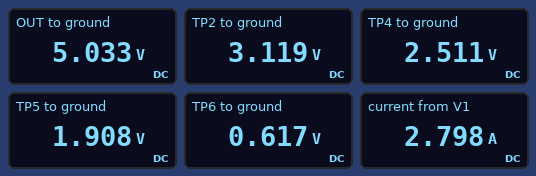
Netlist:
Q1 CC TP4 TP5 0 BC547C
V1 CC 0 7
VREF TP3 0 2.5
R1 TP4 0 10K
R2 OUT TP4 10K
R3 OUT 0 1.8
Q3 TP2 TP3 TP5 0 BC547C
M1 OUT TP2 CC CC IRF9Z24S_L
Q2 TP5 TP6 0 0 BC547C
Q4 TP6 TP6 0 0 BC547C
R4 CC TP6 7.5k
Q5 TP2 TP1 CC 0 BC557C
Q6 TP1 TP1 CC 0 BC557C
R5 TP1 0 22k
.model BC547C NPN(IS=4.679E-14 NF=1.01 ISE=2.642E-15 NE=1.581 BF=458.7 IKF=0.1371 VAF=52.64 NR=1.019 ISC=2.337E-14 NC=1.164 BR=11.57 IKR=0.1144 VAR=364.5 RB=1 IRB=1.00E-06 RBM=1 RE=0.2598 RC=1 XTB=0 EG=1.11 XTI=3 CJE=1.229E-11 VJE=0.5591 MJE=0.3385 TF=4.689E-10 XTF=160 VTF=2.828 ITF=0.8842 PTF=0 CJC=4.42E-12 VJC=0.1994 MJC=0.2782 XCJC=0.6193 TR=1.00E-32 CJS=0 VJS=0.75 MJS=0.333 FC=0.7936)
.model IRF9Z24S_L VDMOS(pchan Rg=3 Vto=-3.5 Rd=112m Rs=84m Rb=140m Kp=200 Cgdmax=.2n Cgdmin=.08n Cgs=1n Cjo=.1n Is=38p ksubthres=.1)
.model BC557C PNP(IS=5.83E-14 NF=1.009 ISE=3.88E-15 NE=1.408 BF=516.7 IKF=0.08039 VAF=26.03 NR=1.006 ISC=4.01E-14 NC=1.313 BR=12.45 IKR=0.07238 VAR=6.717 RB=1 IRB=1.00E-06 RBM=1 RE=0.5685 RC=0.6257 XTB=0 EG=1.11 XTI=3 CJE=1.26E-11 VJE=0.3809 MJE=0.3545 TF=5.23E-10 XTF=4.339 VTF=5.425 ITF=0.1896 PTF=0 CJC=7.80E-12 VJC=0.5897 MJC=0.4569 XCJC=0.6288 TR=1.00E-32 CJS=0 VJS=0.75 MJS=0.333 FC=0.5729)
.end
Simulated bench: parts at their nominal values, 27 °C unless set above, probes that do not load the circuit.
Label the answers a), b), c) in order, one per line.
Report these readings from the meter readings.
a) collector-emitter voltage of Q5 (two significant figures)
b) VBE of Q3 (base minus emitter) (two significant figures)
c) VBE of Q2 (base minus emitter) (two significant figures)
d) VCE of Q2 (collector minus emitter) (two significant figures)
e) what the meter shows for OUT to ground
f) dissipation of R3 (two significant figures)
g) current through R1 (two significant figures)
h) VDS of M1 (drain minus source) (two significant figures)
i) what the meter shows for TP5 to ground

a) -3.9 V
b) 590 mV
c) 620 mV
d) 1.9 V
e) 5.033 V
f) 14 W
g) 250 µA
h) -2.0 V
i) 1.908 V
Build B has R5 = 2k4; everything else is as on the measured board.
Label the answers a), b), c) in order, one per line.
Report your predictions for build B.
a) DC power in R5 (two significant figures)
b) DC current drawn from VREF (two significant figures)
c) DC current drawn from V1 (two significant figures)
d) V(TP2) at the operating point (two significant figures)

a) 17 mW
b) 1.8 µA
c) 4.4 mA
d) 7.0 V
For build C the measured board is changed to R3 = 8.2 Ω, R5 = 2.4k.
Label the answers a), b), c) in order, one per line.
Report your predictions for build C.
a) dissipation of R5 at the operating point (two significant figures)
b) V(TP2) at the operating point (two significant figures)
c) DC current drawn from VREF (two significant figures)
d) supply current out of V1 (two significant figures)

a) 17 mW
b) 7.0 V
c) 1.8 µA
d) 4.4 mA
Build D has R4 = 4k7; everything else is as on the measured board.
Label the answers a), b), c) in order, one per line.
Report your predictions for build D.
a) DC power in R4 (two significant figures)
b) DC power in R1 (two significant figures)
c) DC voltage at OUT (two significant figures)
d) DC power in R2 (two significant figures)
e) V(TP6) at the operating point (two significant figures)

a) 8.6 mW
b) 640 µW
c) 5.1 V
d) 650 µW
e) 630 mV
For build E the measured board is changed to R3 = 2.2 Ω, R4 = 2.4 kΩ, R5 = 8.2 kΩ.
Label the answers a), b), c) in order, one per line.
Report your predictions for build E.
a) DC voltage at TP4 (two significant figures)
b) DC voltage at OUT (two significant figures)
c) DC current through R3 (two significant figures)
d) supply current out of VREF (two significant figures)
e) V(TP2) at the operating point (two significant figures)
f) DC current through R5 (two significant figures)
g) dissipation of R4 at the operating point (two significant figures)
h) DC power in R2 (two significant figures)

a) 2.5 V
b) 5.1 V
c) 2.3 A
d) 1.9 µA
e) 3.2 V
f) 780 µA
g) 17 mW
h) 650 µW
